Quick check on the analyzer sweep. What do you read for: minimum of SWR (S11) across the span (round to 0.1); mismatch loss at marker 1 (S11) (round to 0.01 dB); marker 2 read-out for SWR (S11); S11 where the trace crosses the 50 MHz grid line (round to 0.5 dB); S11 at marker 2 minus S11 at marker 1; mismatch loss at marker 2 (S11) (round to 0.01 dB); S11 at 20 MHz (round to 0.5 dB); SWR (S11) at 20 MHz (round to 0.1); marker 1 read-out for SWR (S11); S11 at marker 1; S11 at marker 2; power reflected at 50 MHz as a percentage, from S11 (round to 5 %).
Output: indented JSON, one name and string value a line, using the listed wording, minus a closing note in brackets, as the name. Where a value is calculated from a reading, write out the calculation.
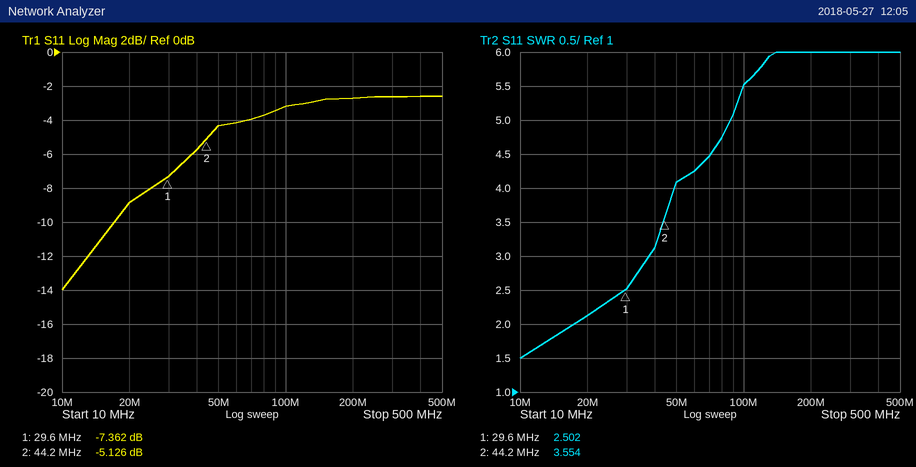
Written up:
{
  "minimum of SWR (S11) across the span": "1.5",
  "mismatch loss at marker 1 (S11)": "−10 log10(1 − 10^(-7.362/10)) ≈ 0.88 dB",
  "marker 2 read-out for SWR": "3.554",
  "S11 where the trace crosses the 50 MHz grid line": "-4.5 dB",
  "S11 at marker 2 minus S11 at marker 1": "-5.126 − (-7.362) = 2.236 dB",
  "mismatch loss at marker 2 (S11)": "−10 log10(1 − 10^(-5.126/10)) ≈ 1.59 dB",
  "S11 at 20 MHz": "-9.0 dB",
  "SWR (S11) at 20 MHz": "2.1",
  "marker 1 read-out for SWR": "2.502",
  "S11 at marker 1": "-7.362 dB",
  "S11 at marker 2": "-5.126 dB",
  "power reflected at 50 MHz as a percentage, from S11": "10^(-4.5/10) ≈ 35 %"
}
